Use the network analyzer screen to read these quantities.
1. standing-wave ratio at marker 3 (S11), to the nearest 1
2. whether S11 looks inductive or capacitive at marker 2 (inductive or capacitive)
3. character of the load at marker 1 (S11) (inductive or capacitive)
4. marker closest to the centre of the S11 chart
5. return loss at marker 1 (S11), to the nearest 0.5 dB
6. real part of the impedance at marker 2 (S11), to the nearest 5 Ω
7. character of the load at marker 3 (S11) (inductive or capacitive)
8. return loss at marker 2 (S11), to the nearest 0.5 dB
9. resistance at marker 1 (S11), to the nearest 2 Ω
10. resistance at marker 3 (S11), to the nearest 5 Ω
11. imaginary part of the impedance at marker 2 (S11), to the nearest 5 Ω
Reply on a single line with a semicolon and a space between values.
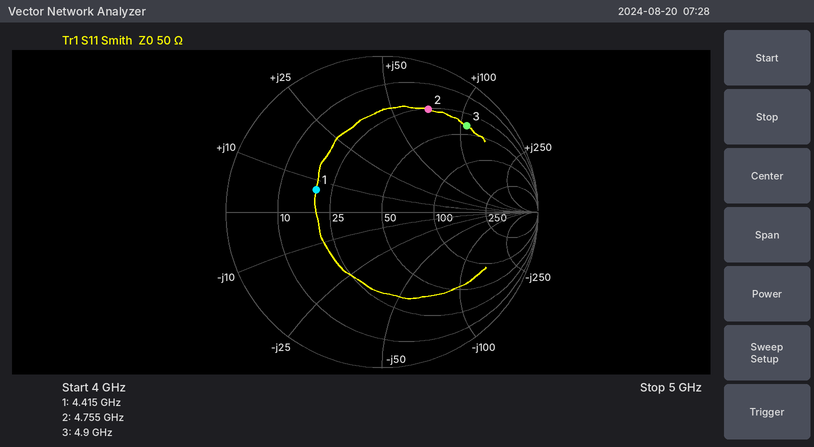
8; inductive; inductive; marker 1; 7.0 dB; 25 Ω; inductive; 3.0 dB; 20 Ω; 40 Ω; +70 Ω
